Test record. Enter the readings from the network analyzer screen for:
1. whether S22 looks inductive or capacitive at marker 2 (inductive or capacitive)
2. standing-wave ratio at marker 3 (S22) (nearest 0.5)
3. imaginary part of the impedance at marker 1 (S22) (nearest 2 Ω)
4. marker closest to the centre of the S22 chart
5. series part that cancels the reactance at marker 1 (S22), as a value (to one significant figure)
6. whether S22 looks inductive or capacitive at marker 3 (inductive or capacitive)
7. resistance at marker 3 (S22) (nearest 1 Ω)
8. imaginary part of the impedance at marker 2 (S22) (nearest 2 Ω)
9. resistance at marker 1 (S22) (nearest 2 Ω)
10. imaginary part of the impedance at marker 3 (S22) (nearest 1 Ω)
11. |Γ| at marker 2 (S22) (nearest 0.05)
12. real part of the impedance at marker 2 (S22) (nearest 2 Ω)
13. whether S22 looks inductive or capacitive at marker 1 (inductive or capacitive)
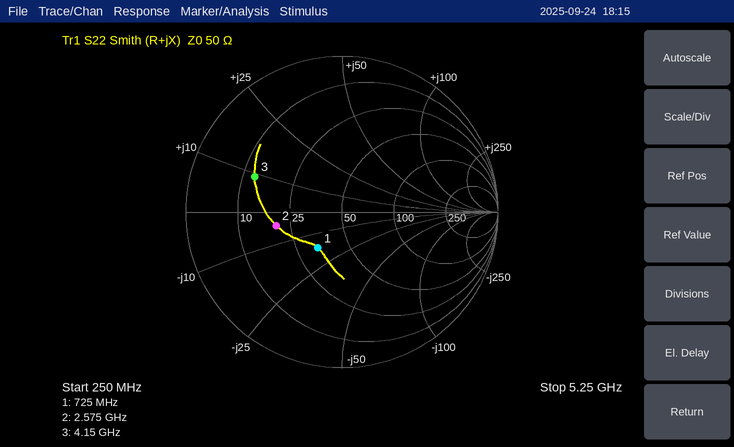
capacitive
4.0
-16 Ω
marker 1
4 nH
inductive
13 Ω
-4 Ω
34 Ω
+9 Ω
0.45
20 Ω
capacitive
